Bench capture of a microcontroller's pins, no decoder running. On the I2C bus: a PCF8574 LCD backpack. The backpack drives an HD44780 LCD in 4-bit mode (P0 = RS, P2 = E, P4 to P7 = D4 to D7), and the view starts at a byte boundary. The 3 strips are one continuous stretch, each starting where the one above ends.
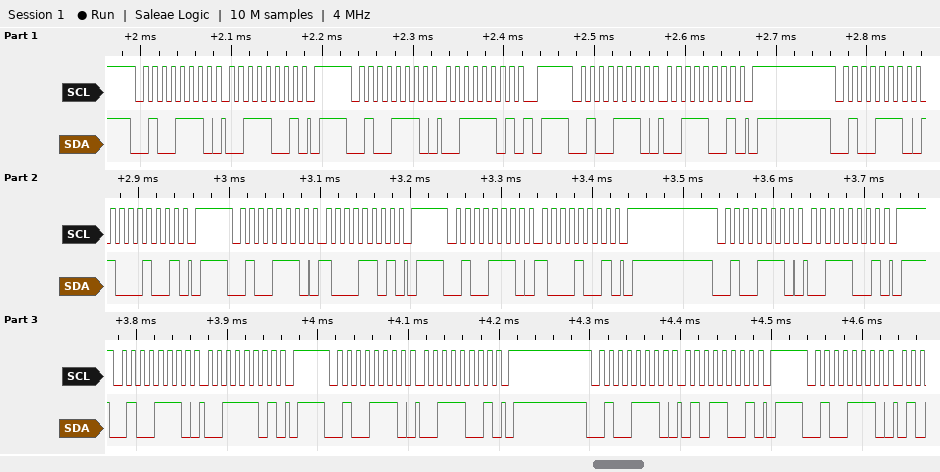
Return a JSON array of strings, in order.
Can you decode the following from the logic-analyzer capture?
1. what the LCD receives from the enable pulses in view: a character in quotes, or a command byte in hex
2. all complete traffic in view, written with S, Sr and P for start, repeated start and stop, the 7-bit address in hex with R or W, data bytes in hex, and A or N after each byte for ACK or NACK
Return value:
["'8'", "S 27W A 39 A P S 27W A 3D A P S 27W A 39 A P S 27W A 89 A P S 27W A 8D A P S 27W A 89 A P S 27W A 39 A P S 27W A 3D A P S 27W A 39 A P S 27W A 59 A P S 27W A"]
